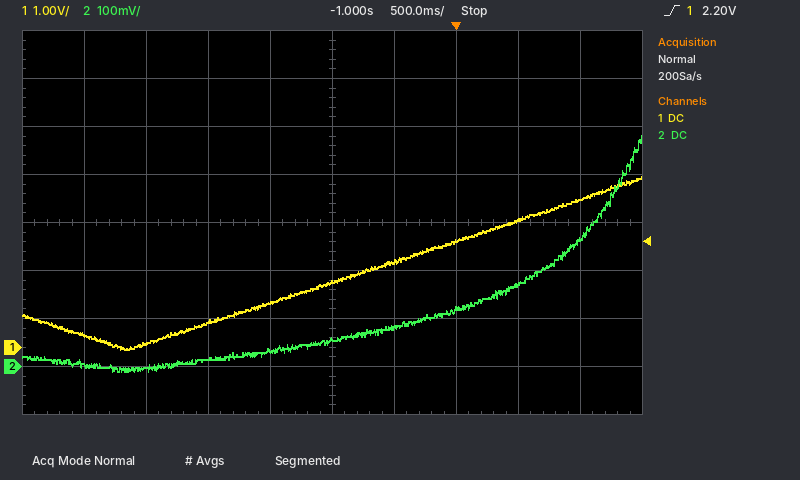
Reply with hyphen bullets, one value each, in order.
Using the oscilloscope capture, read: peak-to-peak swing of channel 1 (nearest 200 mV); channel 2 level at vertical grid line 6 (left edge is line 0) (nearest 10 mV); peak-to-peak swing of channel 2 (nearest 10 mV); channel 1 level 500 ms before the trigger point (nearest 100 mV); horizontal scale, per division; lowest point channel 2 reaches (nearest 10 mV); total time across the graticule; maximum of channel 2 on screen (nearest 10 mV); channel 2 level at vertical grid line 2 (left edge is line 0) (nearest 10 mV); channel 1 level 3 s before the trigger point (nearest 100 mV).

- 3.6 V
- 80 mV
- 490 mV
- 1.8 V
- 500 ms
- -10 mV
- 5 s
- 480 mV
- -10 mV
- 300 mV
